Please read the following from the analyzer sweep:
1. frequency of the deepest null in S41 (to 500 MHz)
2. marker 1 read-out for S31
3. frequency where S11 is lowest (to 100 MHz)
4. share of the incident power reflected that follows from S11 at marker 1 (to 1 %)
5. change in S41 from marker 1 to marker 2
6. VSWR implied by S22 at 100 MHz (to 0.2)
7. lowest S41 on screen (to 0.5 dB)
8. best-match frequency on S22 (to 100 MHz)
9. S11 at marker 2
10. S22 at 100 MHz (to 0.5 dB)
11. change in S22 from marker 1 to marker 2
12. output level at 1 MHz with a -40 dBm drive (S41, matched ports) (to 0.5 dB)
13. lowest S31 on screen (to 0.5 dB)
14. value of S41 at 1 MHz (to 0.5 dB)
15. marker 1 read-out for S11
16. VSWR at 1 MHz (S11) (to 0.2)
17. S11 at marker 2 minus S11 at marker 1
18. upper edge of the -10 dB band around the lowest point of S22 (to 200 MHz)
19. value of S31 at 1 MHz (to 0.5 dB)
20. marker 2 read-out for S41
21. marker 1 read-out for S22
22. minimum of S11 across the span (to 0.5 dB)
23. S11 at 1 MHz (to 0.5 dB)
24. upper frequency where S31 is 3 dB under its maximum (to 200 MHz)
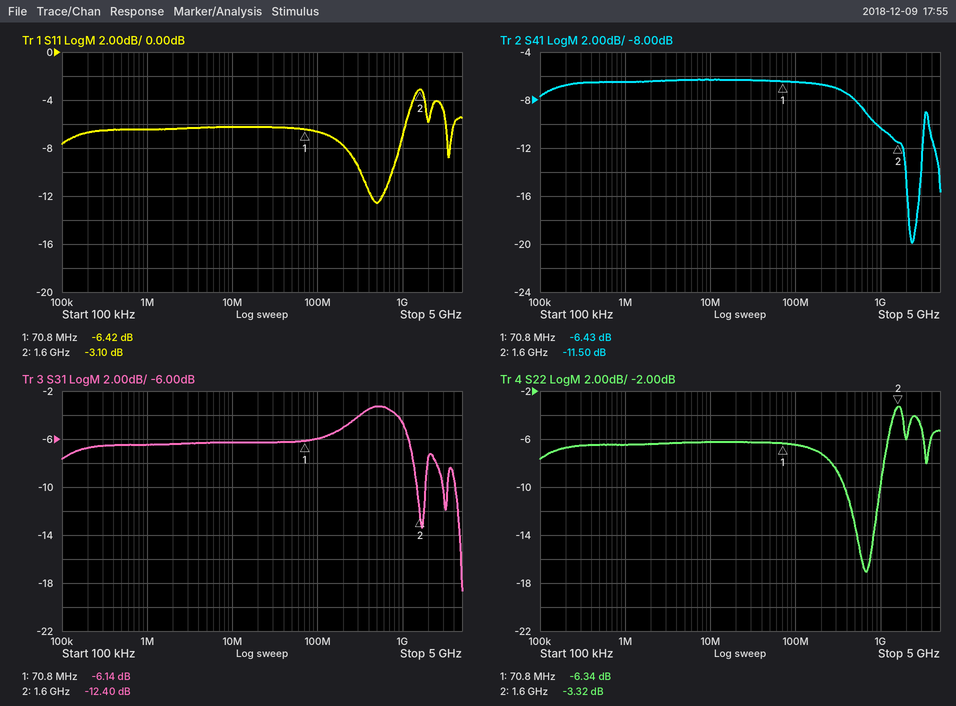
2.5 GHz
-6.14 dB
500 MHz
23 %
-5.07 dB
2.8
-20.0 dB
700 MHz
-3.10 dB
-6.5 dB
3.02 dB
-46.5 dBm
-18.5 dB
-6.5 dB
-6.42 dB
2.8
3.32 dB
1.0 GHz
-6.5 dB
-11.50 dB
-6.34 dB
-12.5 dB
-6.5 dB
1.2 GHz
